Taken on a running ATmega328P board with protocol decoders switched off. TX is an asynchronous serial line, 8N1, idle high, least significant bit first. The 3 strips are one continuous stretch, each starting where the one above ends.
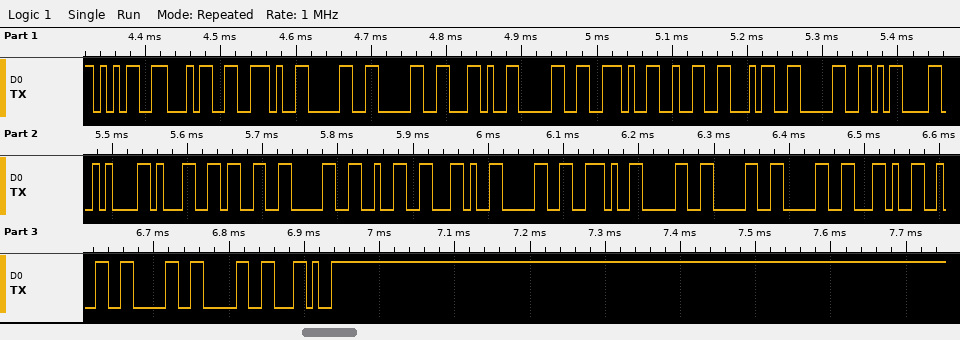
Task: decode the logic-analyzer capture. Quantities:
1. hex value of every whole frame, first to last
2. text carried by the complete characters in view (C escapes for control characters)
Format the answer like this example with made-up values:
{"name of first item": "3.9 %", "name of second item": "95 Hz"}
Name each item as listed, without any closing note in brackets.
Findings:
{"hex value of every whole frame, first to last": "35 34 2E 30 30 2C 30 2E 32 34 30 0D 0A 31 33 30 32 2C 30 2E 30 30 30 2C 32 30 30 2C", "text carried by the complete characters in view": "\"54.00,0.240\\r\\n1302,0.000,200,\""}
